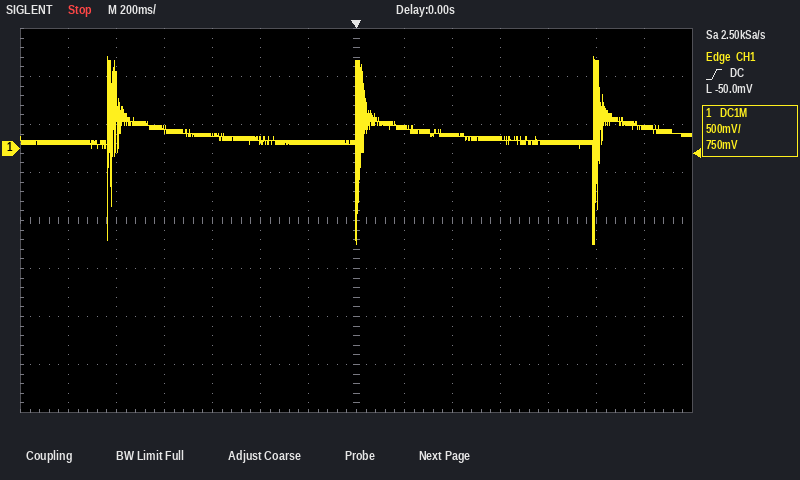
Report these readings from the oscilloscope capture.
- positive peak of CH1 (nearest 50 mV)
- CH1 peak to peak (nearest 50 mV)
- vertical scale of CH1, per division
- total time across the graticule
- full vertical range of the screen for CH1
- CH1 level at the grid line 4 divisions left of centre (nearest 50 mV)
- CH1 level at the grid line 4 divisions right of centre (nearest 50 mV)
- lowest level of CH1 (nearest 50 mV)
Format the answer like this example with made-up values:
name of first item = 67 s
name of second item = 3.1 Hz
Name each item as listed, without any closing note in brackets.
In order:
positive peak of CH1 = 950 mV
CH1 peak to peak = 1.95 V
vertical scale of CH1, per division = 500 mV
total time across the graticule = 2.8 s
full vertical range of the screen for CH1 = 4 V
CH1 level at the grid line 4 divisions left of centre = 200 mV
CH1 level at the grid line 4 divisions right of centre = 50 mV
lowest level of CH1 = -1.00 V
